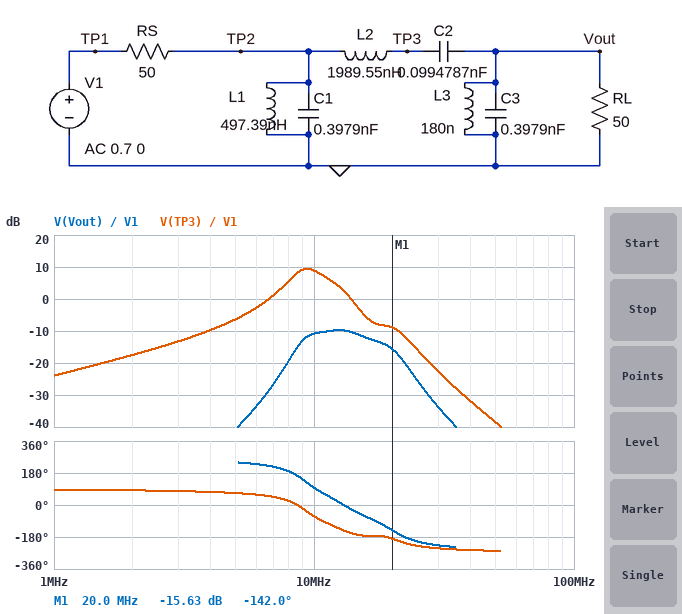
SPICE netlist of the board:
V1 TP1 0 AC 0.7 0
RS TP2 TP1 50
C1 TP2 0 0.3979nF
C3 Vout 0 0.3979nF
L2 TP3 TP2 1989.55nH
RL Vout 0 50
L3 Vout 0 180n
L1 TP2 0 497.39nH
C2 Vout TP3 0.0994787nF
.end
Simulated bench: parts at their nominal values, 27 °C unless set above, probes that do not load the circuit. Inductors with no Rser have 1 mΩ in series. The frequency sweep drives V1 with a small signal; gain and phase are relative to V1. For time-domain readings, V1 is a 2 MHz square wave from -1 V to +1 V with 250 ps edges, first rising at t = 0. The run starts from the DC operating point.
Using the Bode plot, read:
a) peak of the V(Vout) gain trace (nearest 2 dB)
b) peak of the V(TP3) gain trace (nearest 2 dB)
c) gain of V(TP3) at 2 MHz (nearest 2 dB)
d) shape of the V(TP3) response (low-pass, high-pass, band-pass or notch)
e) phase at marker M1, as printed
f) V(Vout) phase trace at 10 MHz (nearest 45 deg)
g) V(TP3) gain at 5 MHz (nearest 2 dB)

-10 dB
10 dB
-18 dB
band-pass
-142.0 deg
90 deg
-6 dB
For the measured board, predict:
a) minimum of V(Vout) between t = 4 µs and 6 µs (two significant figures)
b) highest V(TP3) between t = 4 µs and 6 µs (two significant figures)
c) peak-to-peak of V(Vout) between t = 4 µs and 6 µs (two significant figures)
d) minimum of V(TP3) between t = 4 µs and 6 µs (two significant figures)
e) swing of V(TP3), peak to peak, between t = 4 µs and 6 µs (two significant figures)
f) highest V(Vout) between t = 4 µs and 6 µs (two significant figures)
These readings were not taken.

-160 mV
1.2 V
330 mV
-1.2 V
2.5 V
160 mV
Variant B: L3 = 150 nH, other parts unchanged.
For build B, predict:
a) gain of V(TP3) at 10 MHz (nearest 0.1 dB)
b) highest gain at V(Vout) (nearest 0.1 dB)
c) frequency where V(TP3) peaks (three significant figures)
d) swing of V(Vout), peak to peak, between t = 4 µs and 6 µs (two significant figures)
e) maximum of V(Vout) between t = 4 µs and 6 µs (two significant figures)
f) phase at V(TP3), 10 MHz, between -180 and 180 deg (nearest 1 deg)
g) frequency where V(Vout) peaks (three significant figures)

9.3 dB
-11.2 dB
9.52 MHz
280 mV
140 mV
-60 deg
12.6 MHz
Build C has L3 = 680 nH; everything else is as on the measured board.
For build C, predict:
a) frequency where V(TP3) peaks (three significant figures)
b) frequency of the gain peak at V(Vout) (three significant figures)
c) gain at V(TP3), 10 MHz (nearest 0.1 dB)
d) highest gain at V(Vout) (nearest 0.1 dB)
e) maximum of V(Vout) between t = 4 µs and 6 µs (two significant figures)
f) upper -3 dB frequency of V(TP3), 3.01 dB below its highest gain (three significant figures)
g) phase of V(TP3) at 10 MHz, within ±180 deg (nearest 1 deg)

13.7 MHz
13.0 MHz
4.4 dB
-6.1 dB
250 mV
16.0 MHz
-40 deg
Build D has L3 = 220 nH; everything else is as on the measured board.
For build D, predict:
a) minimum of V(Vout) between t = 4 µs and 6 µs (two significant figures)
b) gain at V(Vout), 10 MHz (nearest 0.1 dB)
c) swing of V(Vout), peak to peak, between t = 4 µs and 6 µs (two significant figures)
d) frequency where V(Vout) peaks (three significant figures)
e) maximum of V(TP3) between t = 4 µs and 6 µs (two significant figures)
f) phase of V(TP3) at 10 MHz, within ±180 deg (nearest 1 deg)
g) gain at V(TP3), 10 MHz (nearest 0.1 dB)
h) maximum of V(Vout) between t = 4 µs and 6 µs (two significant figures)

-190 mV
-9.1 dB
380 mV
12.4 MHz
1.2 V
-66 deg
8.2 dB
190 mV
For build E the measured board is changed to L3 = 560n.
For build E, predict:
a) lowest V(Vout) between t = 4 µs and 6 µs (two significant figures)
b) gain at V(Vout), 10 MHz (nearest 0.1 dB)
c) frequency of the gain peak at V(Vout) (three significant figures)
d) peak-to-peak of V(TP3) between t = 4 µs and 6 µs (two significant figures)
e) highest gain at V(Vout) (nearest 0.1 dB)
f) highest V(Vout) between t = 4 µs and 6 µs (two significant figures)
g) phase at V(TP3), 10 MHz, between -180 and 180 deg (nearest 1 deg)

-250 mV
-6.1 dB
12.8 MHz
2.4 V
-6.0 dB
250 mV
-46 deg
